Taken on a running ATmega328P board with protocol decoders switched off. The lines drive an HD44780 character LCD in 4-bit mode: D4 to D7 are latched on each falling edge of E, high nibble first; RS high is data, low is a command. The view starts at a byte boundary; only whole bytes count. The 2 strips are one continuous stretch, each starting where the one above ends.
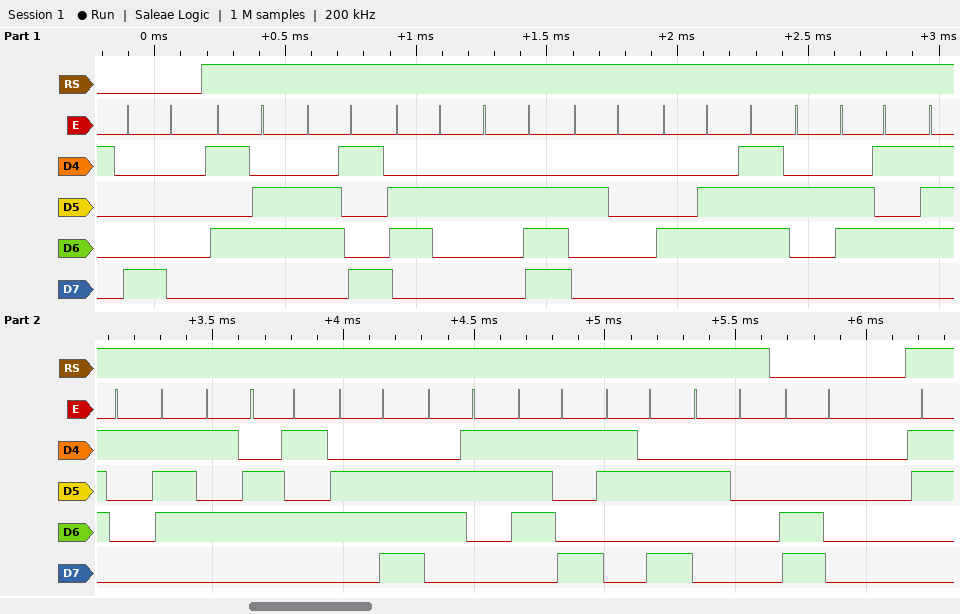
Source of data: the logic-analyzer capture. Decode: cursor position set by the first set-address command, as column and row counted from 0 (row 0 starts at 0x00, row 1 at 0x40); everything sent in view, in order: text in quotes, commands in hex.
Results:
column 0, row 0
0x80 "Vib. Frequency: " 0xC0
